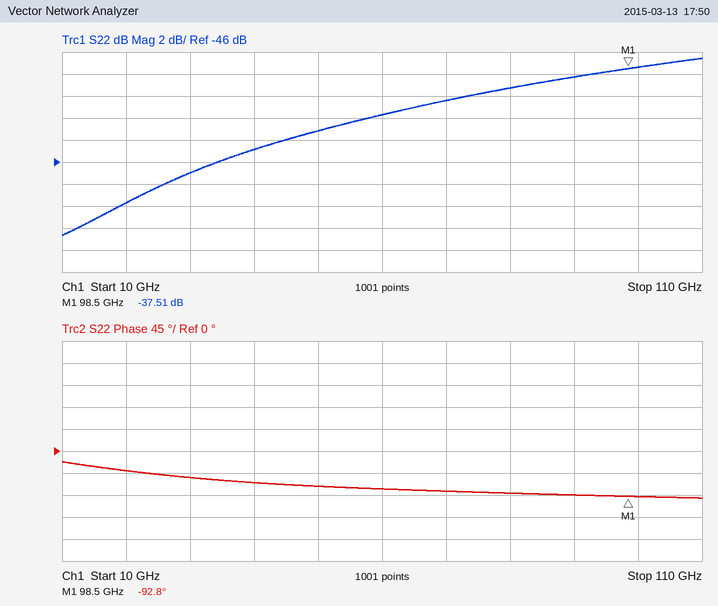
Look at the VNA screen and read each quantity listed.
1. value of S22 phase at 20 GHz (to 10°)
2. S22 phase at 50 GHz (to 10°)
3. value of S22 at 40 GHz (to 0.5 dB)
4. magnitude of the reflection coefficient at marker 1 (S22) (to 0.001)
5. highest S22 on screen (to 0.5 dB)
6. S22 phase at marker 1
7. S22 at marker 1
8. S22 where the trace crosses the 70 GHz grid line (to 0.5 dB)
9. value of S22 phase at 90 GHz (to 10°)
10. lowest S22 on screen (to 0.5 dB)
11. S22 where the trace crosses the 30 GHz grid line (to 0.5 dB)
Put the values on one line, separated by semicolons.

-40°; -70°; -45.0 dB; 0.013; -36.5 dB; -92.8°; -37.51 dB; -40.5 dB; -90°; -52.5 dB; -47.0 dB
